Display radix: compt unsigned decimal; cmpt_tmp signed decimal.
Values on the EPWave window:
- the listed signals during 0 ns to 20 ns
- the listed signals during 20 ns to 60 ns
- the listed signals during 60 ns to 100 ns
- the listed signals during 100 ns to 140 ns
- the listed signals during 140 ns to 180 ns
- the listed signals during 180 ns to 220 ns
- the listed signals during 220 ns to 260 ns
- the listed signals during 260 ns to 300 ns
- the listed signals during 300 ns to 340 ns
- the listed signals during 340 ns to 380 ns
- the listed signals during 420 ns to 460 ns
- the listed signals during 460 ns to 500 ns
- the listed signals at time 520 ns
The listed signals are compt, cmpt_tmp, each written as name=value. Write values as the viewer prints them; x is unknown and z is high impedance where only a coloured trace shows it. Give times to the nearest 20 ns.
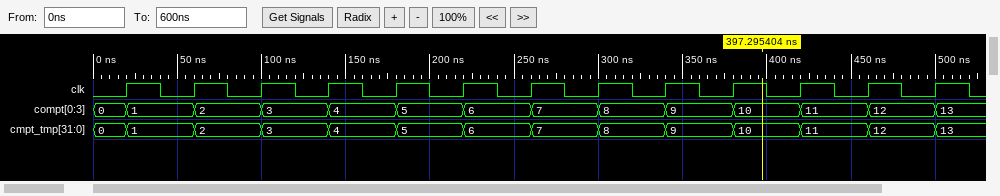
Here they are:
compt=0, cmpt_tmp=0
compt=1, cmpt_tmp=1
compt=2, cmpt_tmp=2
compt=3, cmpt_tmp=3
compt=4, cmpt_tmp=4
compt=5, cmpt_tmp=5
compt=6, cmpt_tmp=6
compt=7, cmpt_tmp=7
compt=8, cmpt_tmp=8
compt=9, cmpt_tmp=9
compt=11, cmpt_tmp=11
compt=12, cmpt_tmp=12
compt=13, cmpt_tmp=13
